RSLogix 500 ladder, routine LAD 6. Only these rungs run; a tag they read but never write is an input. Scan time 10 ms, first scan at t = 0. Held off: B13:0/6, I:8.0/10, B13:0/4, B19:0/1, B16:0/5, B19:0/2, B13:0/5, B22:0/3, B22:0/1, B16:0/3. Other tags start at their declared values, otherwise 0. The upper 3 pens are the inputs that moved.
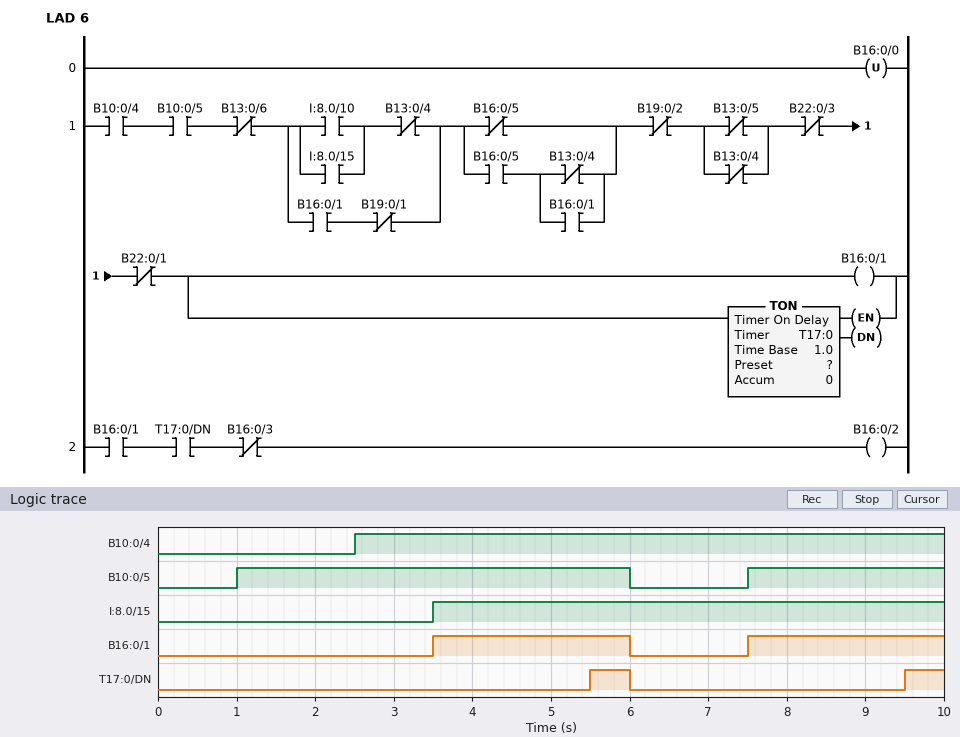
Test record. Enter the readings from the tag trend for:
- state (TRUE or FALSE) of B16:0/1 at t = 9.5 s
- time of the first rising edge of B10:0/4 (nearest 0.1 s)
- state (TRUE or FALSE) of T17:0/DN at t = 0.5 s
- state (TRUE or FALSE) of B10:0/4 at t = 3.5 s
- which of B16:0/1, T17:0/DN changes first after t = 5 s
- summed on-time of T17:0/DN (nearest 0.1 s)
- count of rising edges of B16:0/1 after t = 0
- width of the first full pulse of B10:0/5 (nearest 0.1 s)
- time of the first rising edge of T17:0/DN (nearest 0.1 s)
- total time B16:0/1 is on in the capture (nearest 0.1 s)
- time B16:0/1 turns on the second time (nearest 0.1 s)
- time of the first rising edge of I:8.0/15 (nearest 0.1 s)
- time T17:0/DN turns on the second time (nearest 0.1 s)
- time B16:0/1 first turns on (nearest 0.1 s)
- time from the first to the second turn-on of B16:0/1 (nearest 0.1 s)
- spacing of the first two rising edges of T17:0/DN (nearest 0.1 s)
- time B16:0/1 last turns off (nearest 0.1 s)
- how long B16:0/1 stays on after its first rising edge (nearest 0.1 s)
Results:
TRUE
2.5 s
FALSE
TRUE
T17:0/DN
1.0 s
2
5.0 s
5.5 s
5.0 s
7.5 s
3.5 s
9.5 s
3.5 s
4.0 s
4.0 s
6.0 s
2.5 s
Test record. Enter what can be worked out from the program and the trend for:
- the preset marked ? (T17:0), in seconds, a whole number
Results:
2 s
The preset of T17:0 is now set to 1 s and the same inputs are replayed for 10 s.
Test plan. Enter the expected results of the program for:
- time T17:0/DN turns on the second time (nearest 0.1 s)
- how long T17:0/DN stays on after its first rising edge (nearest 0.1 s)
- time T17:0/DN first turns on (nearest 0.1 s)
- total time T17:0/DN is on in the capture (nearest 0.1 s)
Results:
8.5 s
1.5 s
4.5 s
3.0 s
